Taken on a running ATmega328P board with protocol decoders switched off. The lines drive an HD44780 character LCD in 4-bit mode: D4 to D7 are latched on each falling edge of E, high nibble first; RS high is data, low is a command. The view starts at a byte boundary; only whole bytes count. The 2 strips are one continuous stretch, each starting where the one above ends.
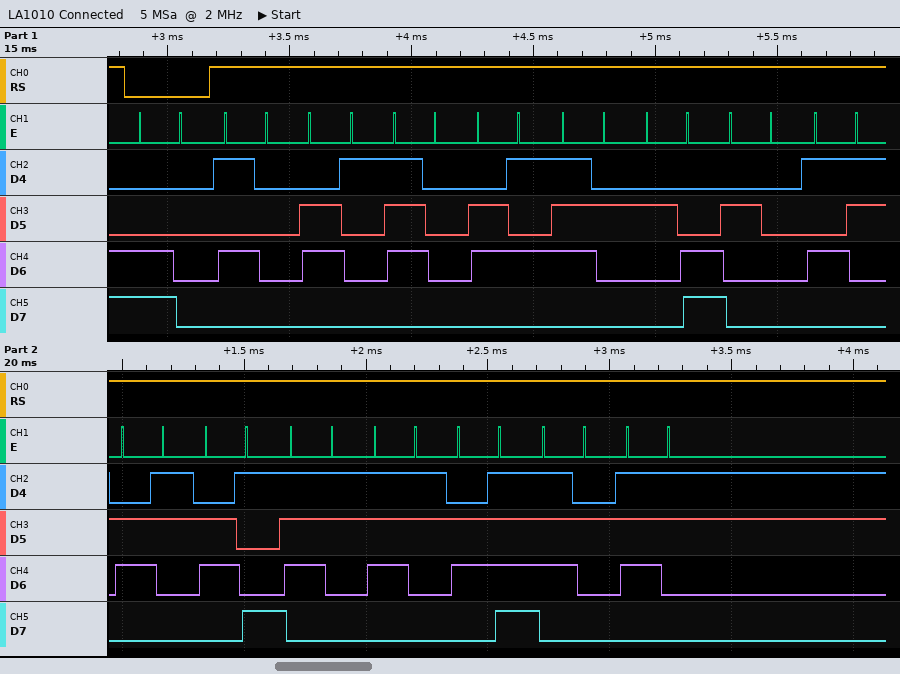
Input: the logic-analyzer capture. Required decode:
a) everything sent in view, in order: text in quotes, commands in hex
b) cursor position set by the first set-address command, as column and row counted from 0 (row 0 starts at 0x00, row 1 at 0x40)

0xC0 "Paper, Scissors"
column 0, row 1
